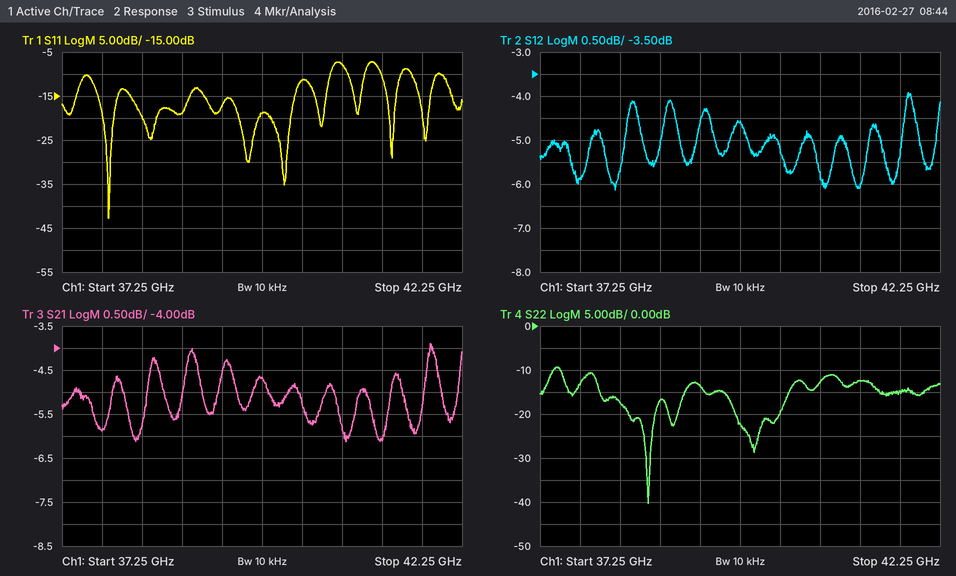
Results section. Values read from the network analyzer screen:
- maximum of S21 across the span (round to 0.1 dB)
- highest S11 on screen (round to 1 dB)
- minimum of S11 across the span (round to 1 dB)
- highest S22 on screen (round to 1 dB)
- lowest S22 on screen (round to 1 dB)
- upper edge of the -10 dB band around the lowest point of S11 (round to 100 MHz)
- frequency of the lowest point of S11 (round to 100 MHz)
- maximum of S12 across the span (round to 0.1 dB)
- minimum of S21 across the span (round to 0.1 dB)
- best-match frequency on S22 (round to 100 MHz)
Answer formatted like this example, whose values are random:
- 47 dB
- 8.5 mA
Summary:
- -3.9 dB
- -7 dB
- -43 dB
- -9 dB
- -40 dB
- 40.6 GHz
- 37.8 GHz
- -3.9 dB
- -6.1 dB
- 38.6 GHz
